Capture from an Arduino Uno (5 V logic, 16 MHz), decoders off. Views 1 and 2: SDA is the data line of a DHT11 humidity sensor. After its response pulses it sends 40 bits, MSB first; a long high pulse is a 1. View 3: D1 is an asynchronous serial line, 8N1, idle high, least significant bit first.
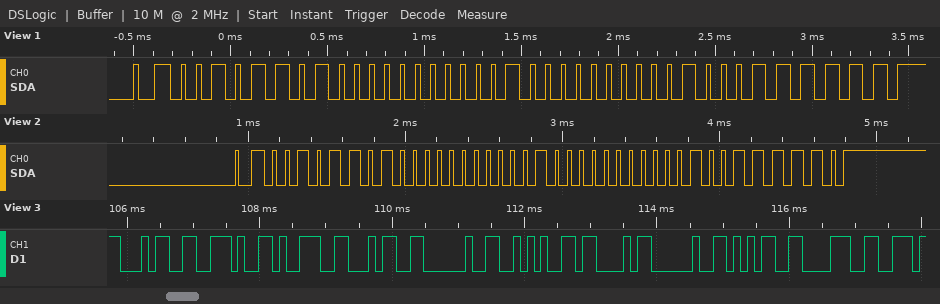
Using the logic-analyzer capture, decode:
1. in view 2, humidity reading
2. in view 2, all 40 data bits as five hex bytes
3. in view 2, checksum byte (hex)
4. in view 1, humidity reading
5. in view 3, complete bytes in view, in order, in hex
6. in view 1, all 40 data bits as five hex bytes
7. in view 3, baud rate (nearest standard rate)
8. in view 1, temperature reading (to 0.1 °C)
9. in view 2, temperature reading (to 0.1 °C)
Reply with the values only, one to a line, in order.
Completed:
45 %
2D 00 10 01 3E
0x3E
45 %
34 2E 39 34 20 2A 43 20 35 38
2D 00 10 02 3F
9600 baud
16.2 °C
16.1 °C
